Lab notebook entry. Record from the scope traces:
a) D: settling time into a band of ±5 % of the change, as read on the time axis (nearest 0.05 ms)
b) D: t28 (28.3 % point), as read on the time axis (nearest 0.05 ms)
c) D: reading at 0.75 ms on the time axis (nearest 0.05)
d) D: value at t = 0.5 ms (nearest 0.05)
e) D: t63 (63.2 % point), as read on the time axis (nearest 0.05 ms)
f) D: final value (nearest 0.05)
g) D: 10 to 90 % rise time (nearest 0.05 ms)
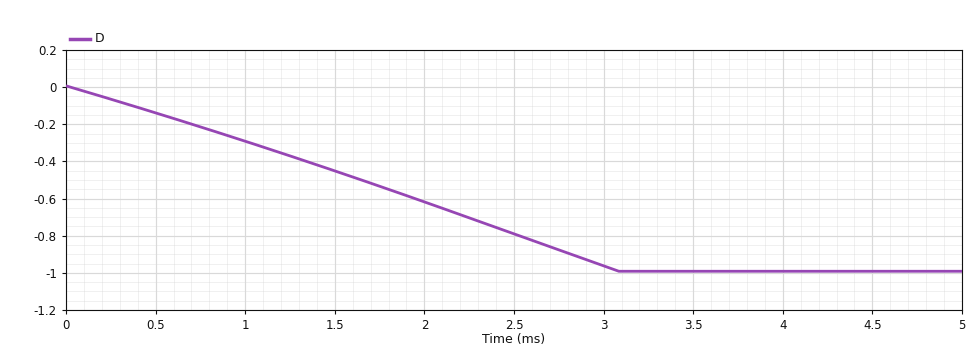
2.95 ms
0.95 ms
-0.20
-0.15
2.00 ms
-1.00
2.45 ms
